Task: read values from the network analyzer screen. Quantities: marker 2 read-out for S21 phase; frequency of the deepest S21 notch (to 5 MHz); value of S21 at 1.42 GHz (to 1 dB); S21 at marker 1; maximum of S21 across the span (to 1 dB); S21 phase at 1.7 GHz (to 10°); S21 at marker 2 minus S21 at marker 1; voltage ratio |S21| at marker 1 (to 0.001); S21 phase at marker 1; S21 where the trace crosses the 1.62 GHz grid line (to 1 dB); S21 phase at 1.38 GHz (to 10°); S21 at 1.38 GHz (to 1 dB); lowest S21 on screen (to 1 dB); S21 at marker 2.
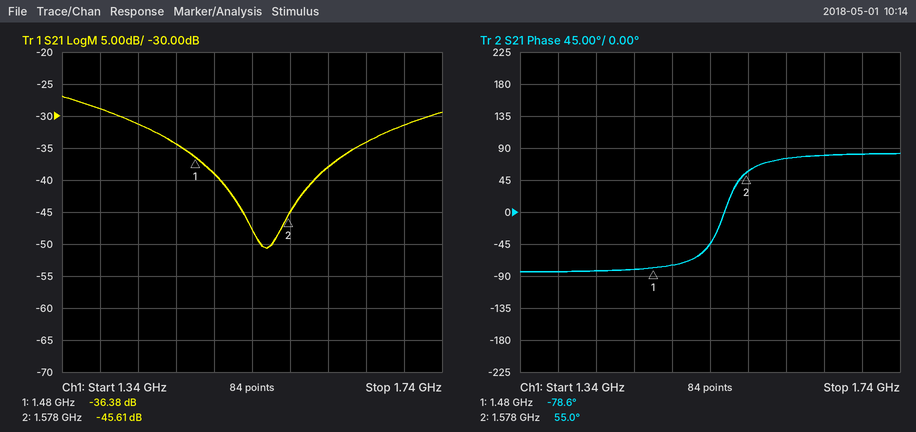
55.0°
1.555 GHz
-31 dB
-36.38 dB
-27 dB
80°
-9.23 dB
0.015
-78.6°
-38 dB
-80°
-29 dB
-51 dB
-45.61 dB
